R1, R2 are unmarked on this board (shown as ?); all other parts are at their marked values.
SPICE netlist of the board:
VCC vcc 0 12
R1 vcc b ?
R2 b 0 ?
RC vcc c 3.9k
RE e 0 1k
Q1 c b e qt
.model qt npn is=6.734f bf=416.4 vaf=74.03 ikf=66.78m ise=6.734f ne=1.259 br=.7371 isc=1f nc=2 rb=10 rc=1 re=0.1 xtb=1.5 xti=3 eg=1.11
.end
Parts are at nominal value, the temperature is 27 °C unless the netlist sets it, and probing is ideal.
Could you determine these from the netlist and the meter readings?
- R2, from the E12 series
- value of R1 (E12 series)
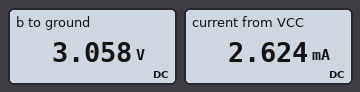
12 kΩ
33 kΩ
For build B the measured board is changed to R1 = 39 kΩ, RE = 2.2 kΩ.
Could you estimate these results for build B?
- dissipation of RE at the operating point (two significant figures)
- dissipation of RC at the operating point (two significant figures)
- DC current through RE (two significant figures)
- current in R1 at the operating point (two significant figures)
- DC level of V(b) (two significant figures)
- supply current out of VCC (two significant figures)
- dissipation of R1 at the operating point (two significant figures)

2.0 mW
3.5 mW
950 µA
240 µA
2.8 V
1.2 mA
2.2 mW
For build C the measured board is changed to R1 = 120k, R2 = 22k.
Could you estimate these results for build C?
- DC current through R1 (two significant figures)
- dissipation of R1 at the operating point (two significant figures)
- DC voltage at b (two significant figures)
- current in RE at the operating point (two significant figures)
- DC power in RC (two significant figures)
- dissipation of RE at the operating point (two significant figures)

86 µA
880 µW
1.7 V
1.1 mA
4.3 mW
1.1 mW
